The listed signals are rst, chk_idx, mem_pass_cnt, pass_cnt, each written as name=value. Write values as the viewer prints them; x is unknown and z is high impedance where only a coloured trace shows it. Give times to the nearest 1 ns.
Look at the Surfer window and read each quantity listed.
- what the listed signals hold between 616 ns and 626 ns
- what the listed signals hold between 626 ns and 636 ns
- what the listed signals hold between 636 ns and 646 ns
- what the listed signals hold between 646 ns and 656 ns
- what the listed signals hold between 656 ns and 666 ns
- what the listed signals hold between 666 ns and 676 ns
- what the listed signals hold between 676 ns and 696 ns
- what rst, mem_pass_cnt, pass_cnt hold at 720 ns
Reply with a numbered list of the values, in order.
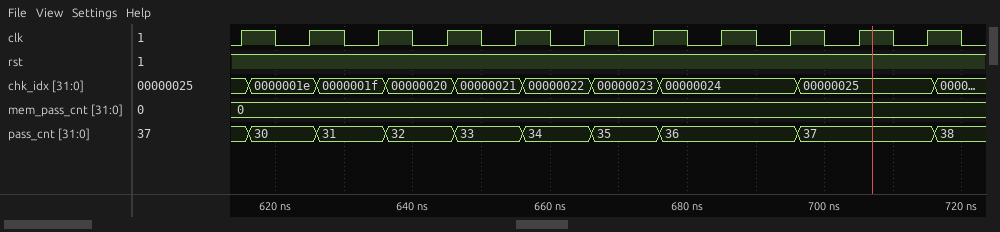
1. rst=1, chk_idx=0000001e, mem_pass_cnt=0, pass_cnt=30
2. rst=1, chk_idx=0000001f, mem_pass_cnt=0, pass_cnt=31
3. rst=1, chk_idx=00000020, mem_pass_cnt=0, pass_cnt=32
4. rst=1, chk_idx=00000021, mem_pass_cnt=0, pass_cnt=33
5. rst=1, chk_idx=00000022, mem_pass_cnt=0, pass_cnt=34
6. rst=1, chk_idx=00000023, mem_pass_cnt=0, pass_cnt=35
7. rst=1, chk_idx=00000024, mem_pass_cnt=0, pass_cnt=36
8. rst=1, mem_pass_cnt=0, pass_cnt=38
